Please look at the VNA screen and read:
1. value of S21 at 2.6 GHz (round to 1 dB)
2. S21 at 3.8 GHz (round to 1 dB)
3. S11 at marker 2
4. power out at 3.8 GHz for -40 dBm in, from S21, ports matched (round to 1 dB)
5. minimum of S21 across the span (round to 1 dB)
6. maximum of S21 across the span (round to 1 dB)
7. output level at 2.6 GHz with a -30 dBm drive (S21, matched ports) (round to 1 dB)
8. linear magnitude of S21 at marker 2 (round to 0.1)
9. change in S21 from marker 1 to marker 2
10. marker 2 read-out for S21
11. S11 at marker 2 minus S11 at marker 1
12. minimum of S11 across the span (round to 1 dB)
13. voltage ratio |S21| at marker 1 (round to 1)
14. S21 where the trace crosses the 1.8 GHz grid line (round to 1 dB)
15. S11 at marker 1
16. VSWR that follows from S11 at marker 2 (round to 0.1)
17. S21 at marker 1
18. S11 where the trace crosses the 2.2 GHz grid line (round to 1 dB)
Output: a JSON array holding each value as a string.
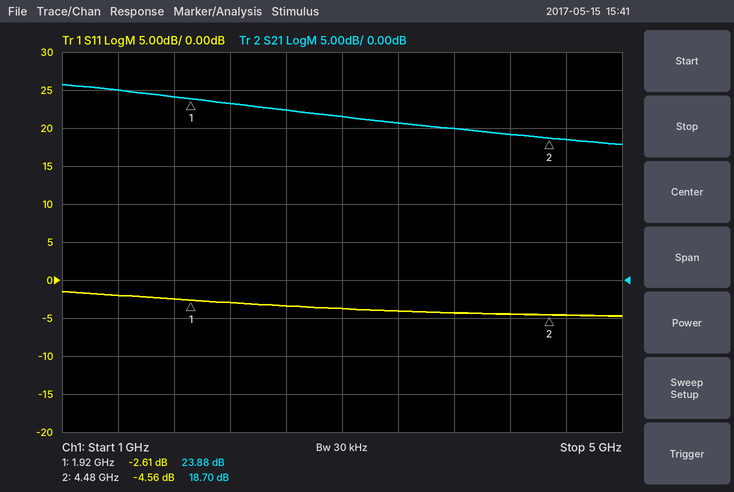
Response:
["22 dB", "20 dB", "-4.56 dB", "-20 dBm", "18 dB", "26 dB", "-8 dBm", "8.6", "-5.18 dB", "18.70 dB", "-1.95 dB", "-5 dB", "16", "24 dB", "-2.61 dB", "3.9", "23.88 dB", "-3 dB"]
